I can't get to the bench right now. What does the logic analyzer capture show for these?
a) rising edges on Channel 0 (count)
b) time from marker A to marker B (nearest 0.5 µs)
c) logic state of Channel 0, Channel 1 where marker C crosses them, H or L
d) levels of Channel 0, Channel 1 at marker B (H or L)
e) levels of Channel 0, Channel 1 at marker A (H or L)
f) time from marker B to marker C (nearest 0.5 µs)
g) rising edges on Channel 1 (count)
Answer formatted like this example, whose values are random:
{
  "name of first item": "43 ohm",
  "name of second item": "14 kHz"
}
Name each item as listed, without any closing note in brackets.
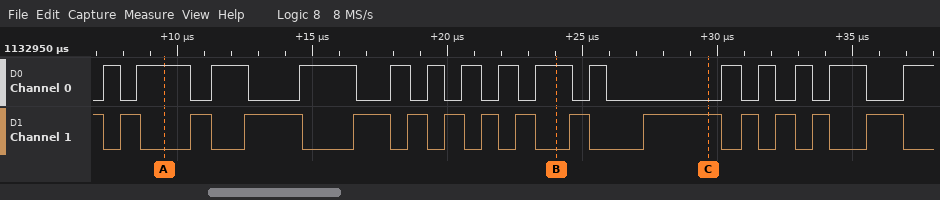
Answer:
{
  "rising edges on Channel 0": "15",
  "time from marker A to marker B": "14.5 µs",
  "logic state of Channel 0, Channel 1 where marker C crosses them, H or L": "Channel 0=L, Channel 1=H",
  "levels of Channel 0, Channel 1 at marker B": "Channel 0=H, Channel 1=L",
  "levels of Channel 0, Channel 1 at marker A": "Channel 0=H, Channel 1=L",
  "time from marker B to marker C": "5.5 µs",
  "rising edges on Channel 1": "14"
}
